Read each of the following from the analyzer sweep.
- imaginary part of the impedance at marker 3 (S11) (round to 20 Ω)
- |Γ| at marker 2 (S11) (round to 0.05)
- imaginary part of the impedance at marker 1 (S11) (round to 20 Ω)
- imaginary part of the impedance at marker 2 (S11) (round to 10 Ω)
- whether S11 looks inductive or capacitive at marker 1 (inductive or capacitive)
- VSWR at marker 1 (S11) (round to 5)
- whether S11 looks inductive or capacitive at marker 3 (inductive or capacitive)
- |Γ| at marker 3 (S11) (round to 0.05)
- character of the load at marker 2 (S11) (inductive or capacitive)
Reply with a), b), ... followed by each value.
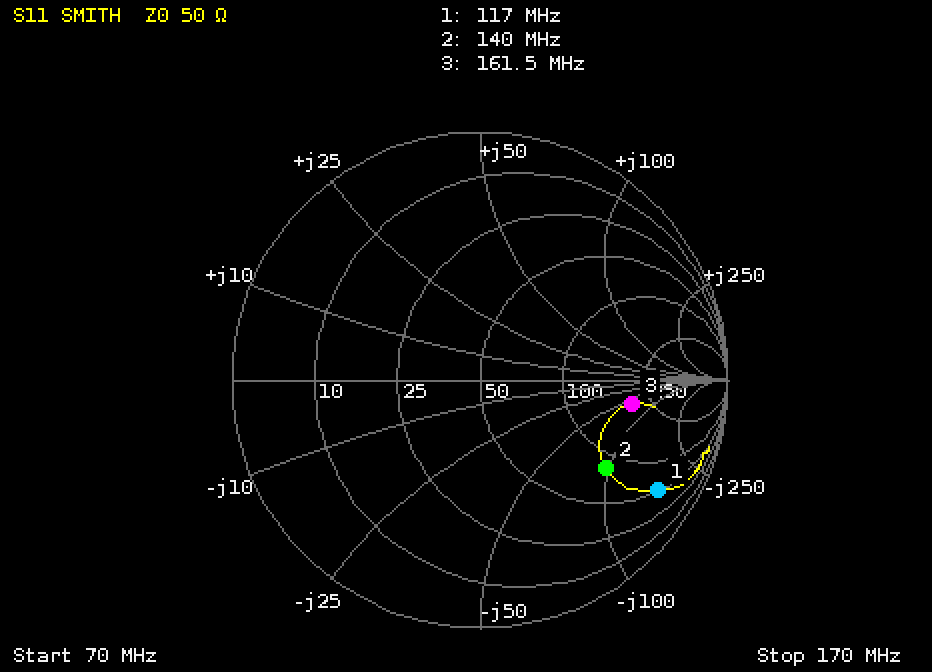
a) -60 Ω
b) 0.60
c) -160 Ω
d) -100 Ω
e) capacitive
f) 10
g) capacitive
h) 0.60
i) capacitive
